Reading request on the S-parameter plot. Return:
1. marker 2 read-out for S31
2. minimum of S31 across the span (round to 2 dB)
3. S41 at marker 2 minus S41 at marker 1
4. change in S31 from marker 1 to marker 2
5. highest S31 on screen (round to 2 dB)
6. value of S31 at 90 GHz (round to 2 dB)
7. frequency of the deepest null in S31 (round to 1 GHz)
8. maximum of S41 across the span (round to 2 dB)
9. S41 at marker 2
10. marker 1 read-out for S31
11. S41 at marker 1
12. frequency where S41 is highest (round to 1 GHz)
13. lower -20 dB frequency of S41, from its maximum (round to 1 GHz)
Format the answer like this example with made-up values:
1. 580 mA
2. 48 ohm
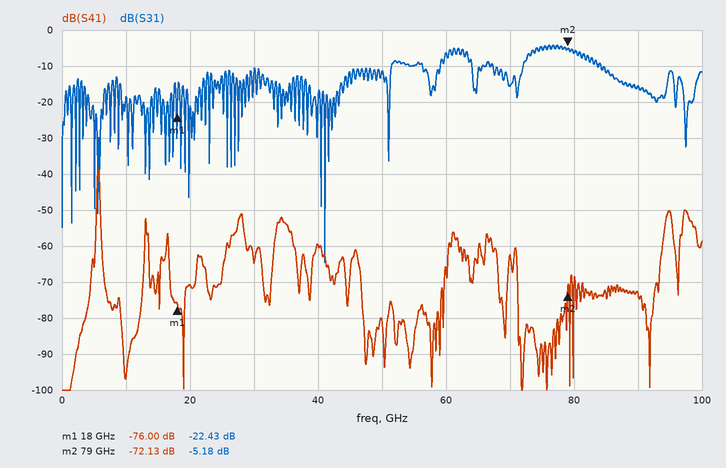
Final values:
1. -5.18 dB
2. -64 dB
3. 3.87 dB
4. 17.25 dB
5. -4 dB
6. -16 dB
7. 41 GHz
8. -38 dB
9. -72.13 dB
10. -22.43 dB
11. -76.00 dB
12. 6 GHz
13. 5 GHz
